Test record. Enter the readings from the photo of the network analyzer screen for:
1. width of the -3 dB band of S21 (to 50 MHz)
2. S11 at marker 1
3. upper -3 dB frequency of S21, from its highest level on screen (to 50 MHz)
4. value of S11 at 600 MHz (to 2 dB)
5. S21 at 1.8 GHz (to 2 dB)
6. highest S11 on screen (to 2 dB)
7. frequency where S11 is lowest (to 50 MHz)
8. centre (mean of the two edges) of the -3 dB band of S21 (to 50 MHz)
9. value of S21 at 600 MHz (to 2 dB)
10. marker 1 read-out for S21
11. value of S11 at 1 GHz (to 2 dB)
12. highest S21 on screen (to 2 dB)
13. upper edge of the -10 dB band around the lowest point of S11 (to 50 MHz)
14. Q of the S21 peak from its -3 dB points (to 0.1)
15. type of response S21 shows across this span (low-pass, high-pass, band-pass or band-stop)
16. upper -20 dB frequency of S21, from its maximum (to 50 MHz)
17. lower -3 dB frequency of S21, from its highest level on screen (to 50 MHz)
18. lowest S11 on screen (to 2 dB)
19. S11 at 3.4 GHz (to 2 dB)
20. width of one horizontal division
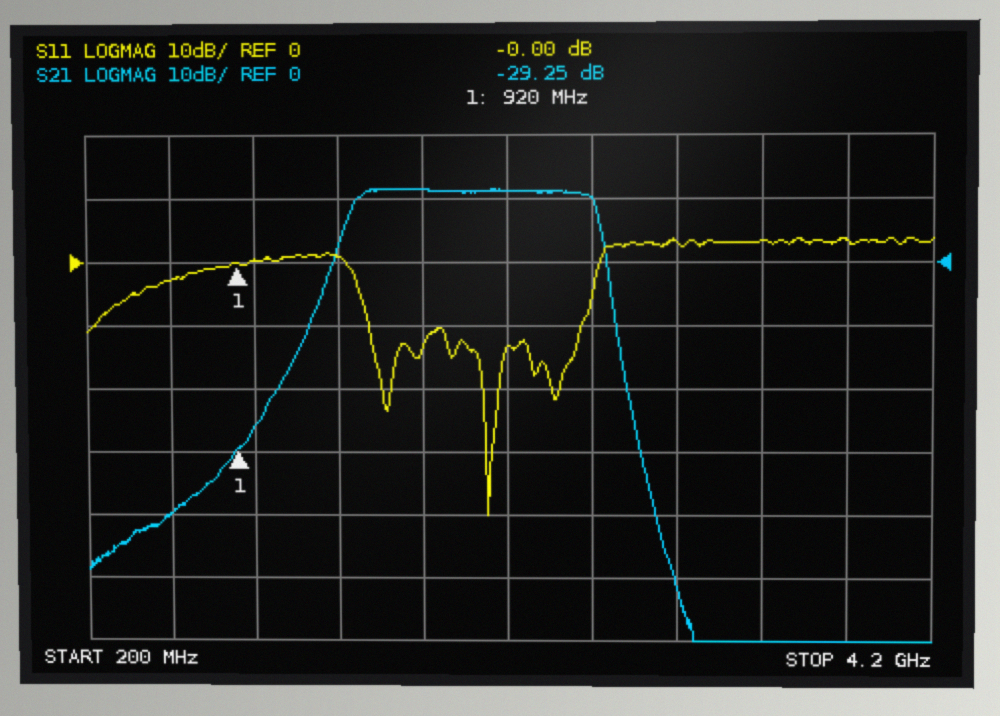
1.15 GHz
-0.00 dB
2.60 GHz
-2 dB
12 dB
4 dB
2.10 GHz
2.05 GHz
-40 dB
-29.25 dB
0 dB
12 dB
2.55 GHz
1.8
band-pass
2.70 GHz
1.45 GHz
-40 dB
4 dB
400 MHz
